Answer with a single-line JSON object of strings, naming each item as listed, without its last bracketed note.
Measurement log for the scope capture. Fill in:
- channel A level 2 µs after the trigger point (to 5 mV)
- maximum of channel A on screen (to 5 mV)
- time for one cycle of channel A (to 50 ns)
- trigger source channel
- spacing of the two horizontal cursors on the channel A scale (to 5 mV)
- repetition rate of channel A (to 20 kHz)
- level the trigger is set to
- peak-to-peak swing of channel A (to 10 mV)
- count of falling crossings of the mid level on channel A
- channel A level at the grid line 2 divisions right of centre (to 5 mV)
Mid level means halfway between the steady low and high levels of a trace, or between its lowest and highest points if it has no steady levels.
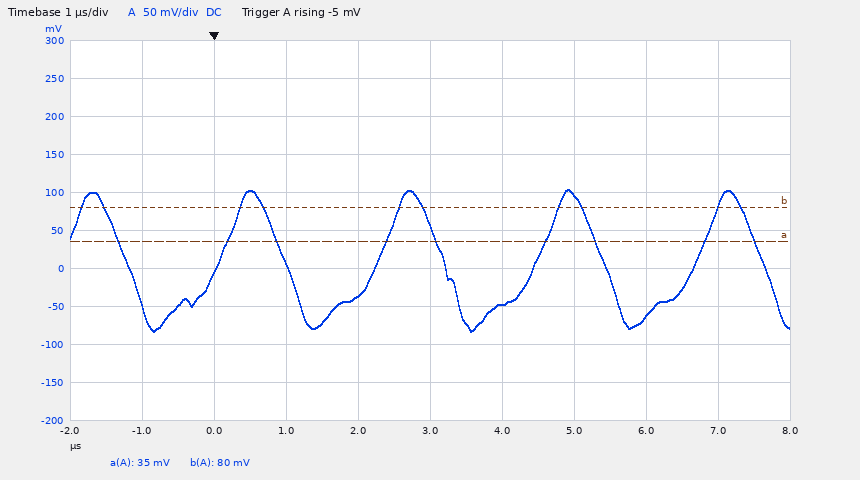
{"channel A level 2 µs after the trigger point": "-35 mV", "maximum of channel A on screen": "105 mV", "time for one cycle of channel A": "2.20 µs", "trigger source channel": "channel A", "spacing of the two horizontal cursors on the channel A scale": "45 mV", "repetition rate of channel A": "460 kHz", "level the trigger is set to": "-5 mV", "peak-to-peak swing of channel A": "190 mV", "count of falling crossings of the mid level on channel A": "5", "channel A level at the grid line 2 divisions right of centre": "95 mV"}
